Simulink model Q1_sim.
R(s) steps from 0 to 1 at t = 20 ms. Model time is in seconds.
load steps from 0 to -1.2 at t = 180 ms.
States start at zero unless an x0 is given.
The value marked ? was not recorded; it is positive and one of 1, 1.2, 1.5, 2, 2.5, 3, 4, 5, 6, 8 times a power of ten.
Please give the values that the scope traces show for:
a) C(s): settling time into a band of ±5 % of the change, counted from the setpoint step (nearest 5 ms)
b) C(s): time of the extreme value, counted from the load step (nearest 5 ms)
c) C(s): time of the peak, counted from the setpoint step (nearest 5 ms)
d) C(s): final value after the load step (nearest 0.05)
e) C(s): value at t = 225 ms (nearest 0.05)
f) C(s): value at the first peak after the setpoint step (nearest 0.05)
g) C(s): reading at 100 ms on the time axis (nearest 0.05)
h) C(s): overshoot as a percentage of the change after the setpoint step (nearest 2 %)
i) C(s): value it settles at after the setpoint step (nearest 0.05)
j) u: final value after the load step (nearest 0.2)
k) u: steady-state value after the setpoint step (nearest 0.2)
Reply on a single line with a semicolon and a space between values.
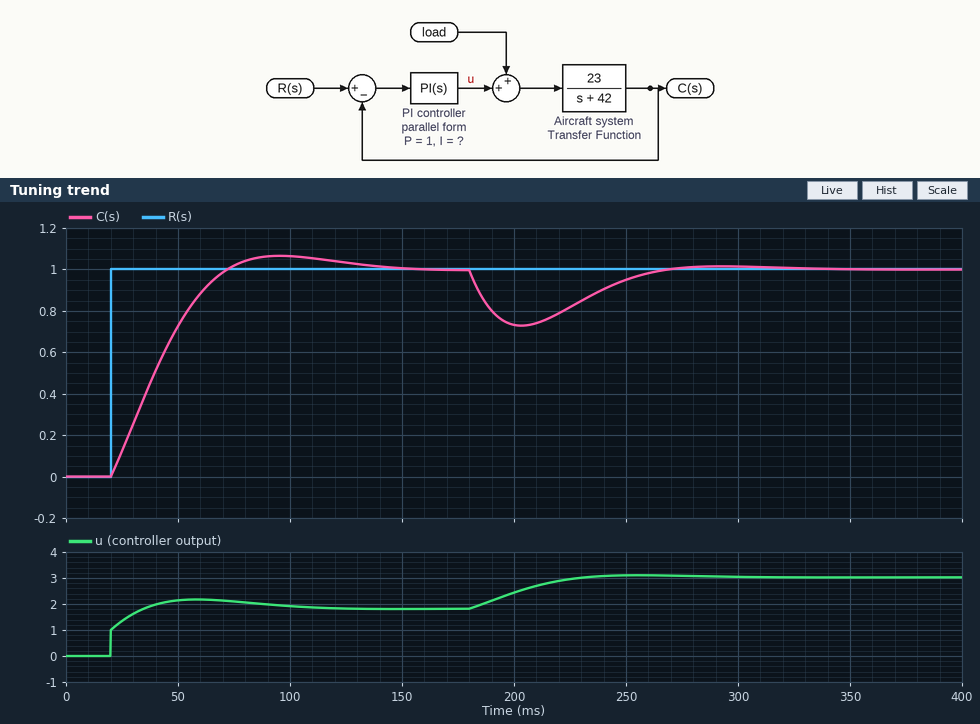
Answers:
95 ms; 25 ms; 75 ms; 1.00; 0.80; 1.05; 1.05; 6 %; 1.00; 3.0; 1.8
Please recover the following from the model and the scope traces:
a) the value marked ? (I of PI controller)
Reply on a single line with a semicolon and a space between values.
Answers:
100
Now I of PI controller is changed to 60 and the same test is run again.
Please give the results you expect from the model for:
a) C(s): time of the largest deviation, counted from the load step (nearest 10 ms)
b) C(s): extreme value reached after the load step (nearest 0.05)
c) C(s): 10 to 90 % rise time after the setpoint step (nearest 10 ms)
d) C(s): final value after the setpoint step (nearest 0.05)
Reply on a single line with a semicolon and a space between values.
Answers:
30 ms; 0.70; 60 ms; 1.00
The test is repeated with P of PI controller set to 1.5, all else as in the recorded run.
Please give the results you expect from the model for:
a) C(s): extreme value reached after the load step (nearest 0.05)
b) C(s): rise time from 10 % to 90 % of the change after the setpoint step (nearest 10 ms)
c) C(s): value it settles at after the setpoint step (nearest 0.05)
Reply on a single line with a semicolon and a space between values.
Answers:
0.75; 40 ms; 1.00
